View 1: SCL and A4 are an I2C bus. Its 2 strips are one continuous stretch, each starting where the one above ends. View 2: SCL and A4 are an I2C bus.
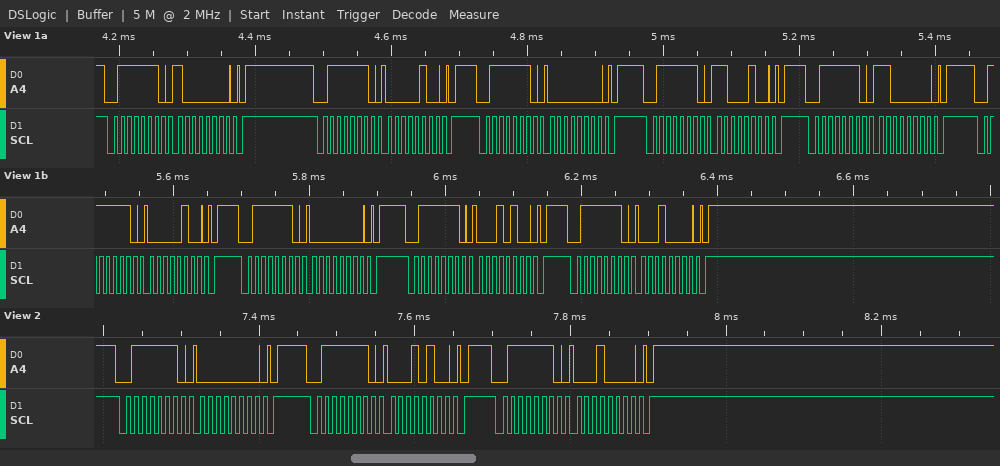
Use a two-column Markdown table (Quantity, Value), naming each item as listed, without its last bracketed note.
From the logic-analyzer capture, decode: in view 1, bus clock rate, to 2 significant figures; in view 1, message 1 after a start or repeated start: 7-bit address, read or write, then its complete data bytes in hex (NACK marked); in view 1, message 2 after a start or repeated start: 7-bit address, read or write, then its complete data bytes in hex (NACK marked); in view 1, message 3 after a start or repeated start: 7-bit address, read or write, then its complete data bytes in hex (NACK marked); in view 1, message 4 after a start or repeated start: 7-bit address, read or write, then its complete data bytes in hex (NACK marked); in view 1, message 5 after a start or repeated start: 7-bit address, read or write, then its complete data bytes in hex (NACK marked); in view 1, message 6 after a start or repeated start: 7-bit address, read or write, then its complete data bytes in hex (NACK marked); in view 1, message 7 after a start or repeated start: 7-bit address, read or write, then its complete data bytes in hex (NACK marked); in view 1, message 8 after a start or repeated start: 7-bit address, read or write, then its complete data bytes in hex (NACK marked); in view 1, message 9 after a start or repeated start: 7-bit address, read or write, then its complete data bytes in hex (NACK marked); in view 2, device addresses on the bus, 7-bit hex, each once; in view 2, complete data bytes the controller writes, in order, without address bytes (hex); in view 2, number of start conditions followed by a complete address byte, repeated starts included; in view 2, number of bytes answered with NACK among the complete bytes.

| Quantity | Value |
|---|---|
| in view 1, bus clock rate, to 2 significant figures | 100 kHz |
| in view 1, message 1 after a start or repeated start: 7-bit address, read or write, then its complete data bytes in hex | 0x3F write: 80 |
| in view 1, message 2 after a start or repeated start: 7-bit address, read or write, then its complete data bytes in hex | 0x3F write: 04 |
| in view 1, message 3 after a start or repeated start: 7-bit address, read or write, then its complete data bytes in hex | 0x3F write: 00 |
| in view 1, message 4 after a start or repeated start: 7-bit address, read or write, then its complete data bytes in hex | 0x3F write: C4 |
| in view 1, message 5 after a start or repeated start: 7-bit address, read or write, then its complete data bytes in hex | 0x3F write: C0 |
| in view 1, message 6 after a start or repeated start: 7-bit address, read or write, then its complete data bytes in hex | 0x3F write: 04 |
| in view 1, message 7 after a start or repeated start: 7-bit address, read or write, then its complete data bytes in hex | 0x3F write: 00 |
| in view 1, message 8 after a start or repeated start: 7-bit address, read or write, then its complete data bytes in hex | 0x3F write: 14 |
| in view 1, message 9 after a start or repeated start: 7-bit address, read or write, then its complete data bytes in hex | 0x3F write: 10 |
| in view 2, device addresses on the bus, 7-bit hex, each once | 0x3F |
| in view 2, complete data bytes the controller writes, in order, without address bytes | 00 14 10 |
| in view 2, number of start conditions followed by a complete address byte, repeated starts included | 3 |
| in view 2, number of bytes answered with NACK among the complete bytes | 0 |
